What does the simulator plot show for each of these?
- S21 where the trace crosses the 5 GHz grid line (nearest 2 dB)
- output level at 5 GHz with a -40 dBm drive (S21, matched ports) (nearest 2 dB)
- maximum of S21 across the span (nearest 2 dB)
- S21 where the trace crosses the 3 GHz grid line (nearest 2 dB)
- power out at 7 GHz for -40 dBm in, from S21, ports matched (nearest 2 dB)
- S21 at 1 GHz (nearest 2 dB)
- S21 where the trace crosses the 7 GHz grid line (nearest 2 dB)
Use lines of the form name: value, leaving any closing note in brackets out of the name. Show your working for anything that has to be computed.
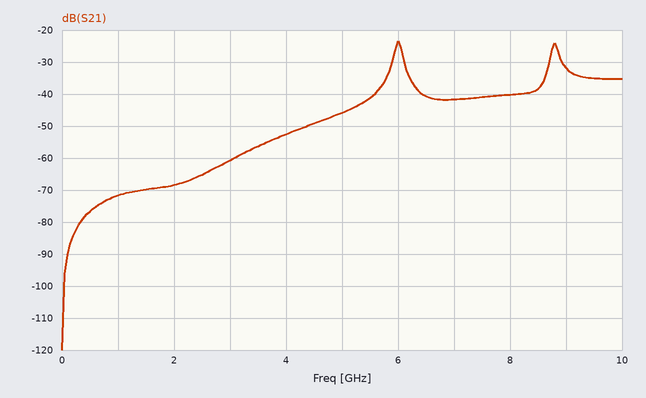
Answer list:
S21 where the trace crosses the 5 GHz grid line: -46 dB
output level at 5 GHz with a -40 dBm drive (S21, matched ports): -40 dBm + (-46 dB) = -86 dBm
maximum of S21 across the span: -24 dB
S21 where the trace crosses the 3 GHz grid line: -60 dB
power out at 7 GHz for -40 dBm in, from S21, ports matched: -40 dBm + (-42 dB) = -82 dBm
S21 at 1 GHz: -72 dB
S21 where the trace crosses the 7 GHz grid line: -42 dB
